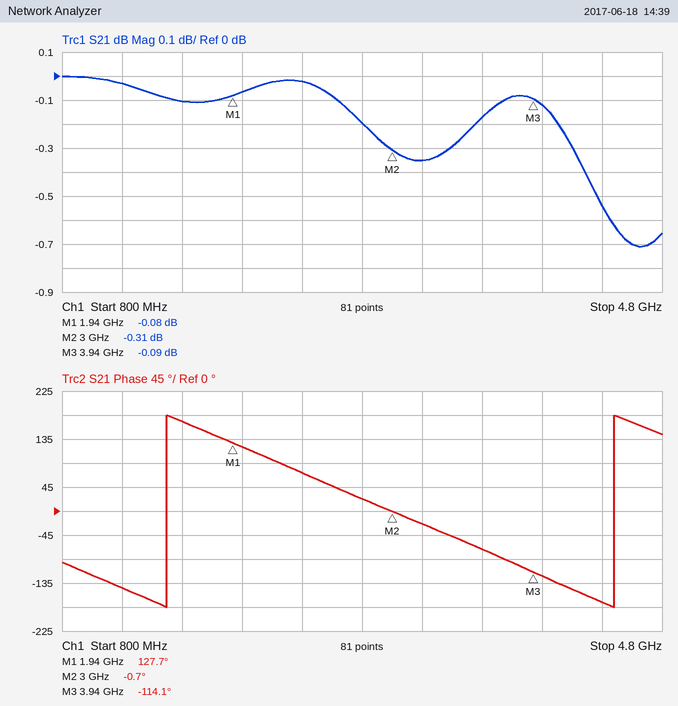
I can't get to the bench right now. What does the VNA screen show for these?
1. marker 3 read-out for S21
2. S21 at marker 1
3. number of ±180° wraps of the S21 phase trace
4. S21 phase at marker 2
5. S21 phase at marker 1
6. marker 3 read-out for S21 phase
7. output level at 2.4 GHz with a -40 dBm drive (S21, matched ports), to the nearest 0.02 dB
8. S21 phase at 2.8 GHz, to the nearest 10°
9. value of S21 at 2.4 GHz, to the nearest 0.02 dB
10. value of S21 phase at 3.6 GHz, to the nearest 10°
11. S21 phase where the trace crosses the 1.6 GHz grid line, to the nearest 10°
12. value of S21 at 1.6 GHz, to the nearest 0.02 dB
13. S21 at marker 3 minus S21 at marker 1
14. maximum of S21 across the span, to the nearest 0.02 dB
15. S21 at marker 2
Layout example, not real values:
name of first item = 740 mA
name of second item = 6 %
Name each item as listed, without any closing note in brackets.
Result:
marker 3 read-out for S21 = -0.09 dB
S21 at marker 1 = -0.08 dB
number of ±180° wraps of the S21 phase trace = 2
S21 phase at marker 2 = -0.7°
S21 phase at marker 1 = 127.7°
marker 3 read-out for S21 phase = -114.1°
output level at 2.4 GHz with a -40 dBm drive (S21, matched ports), to the nearest 0.02 dB = -40.02 dBm
S21 phase at 2.8 GHz, to the nearest 10° = 20°
value of S21 at 2.4 GHz, to the nearest 0.02 dB = -0.02 dB
value of S21 phase at 3.6 GHz, to the nearest 10° = -70°
S21 phase where the trace crosses the 1.6 GHz grid line, to the nearest 10° = 170°
value of S21 at 1.6 GHz, to the nearest 0.02 dB = -0.10 dB
S21 at marker 3 minus S21 at marker 1 = -0.01 dB
maximum of S21 across the span, to the nearest 0.02 dB = 0.00 dB
S21 at marker 2 = -0.31 dB
